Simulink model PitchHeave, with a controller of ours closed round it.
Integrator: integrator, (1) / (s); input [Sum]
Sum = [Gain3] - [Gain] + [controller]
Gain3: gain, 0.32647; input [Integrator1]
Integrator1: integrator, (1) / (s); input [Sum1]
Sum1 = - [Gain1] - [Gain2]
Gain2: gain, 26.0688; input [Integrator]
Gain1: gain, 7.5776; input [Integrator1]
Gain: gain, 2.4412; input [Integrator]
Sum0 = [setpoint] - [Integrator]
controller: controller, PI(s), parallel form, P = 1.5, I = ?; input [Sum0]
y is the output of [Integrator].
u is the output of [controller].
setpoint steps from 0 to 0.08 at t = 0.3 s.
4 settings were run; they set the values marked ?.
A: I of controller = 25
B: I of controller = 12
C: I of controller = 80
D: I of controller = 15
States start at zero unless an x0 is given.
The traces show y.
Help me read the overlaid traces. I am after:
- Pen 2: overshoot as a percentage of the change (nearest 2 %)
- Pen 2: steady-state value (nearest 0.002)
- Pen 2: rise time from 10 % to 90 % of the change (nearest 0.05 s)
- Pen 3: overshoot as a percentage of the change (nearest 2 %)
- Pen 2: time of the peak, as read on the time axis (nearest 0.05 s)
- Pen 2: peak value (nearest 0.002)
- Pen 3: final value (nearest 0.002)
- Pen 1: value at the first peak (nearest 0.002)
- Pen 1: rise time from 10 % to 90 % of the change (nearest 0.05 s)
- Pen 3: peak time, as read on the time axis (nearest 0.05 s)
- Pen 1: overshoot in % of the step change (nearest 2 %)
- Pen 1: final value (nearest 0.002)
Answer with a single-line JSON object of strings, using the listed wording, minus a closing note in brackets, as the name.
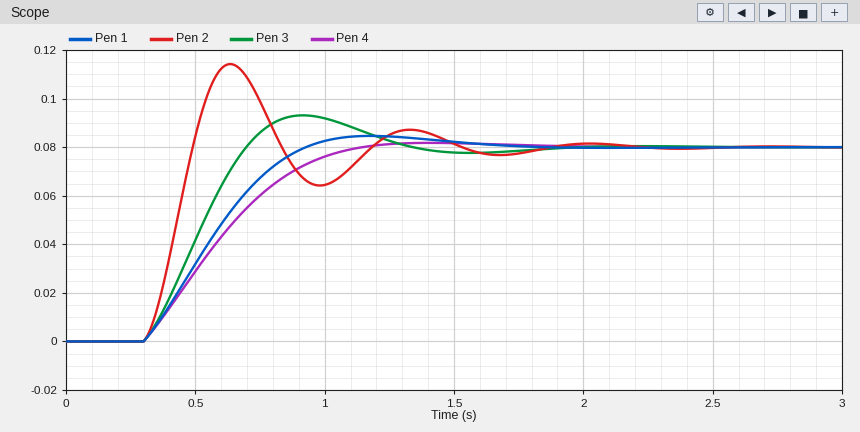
{"Pen 2: overshoot as a percentage of the change": "42 %", "Pen 2: steady-state value": "0.080", "Pen 2: rise time from 10 % to 90 % of the change": "0.15 s", "Pen 3: overshoot as a percentage of the change": "16 %", "Pen 2: time of the peak, as read on the time axis": "0.65 s", "Pen 2: peak value": "0.114", "Pen 3: final value": "0.080", "Pen 1: value at the first peak": "0.084", "Pen 1: rise time from 10 % to 90 % of the change": "0.45 s", "Pen 3: peak time, as read on the time axis": "0.90 s", "Pen 1: overshoot in % of the step change": "6 %", "Pen 1: final value": "0.080"}
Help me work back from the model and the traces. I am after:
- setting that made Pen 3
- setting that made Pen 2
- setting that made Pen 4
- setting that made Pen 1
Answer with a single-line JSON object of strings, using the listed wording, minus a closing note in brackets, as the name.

{"setting that made Pen 3": "A", "setting that made Pen 2": "C", "setting that made Pen 4": "B", "setting that made Pen 1": "D"}
